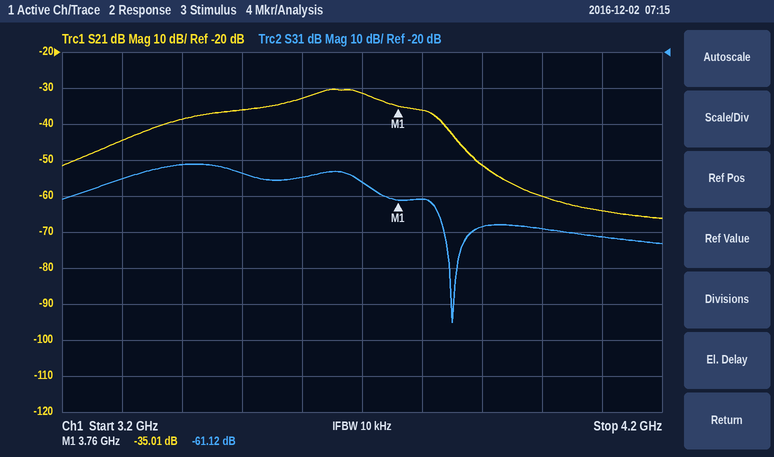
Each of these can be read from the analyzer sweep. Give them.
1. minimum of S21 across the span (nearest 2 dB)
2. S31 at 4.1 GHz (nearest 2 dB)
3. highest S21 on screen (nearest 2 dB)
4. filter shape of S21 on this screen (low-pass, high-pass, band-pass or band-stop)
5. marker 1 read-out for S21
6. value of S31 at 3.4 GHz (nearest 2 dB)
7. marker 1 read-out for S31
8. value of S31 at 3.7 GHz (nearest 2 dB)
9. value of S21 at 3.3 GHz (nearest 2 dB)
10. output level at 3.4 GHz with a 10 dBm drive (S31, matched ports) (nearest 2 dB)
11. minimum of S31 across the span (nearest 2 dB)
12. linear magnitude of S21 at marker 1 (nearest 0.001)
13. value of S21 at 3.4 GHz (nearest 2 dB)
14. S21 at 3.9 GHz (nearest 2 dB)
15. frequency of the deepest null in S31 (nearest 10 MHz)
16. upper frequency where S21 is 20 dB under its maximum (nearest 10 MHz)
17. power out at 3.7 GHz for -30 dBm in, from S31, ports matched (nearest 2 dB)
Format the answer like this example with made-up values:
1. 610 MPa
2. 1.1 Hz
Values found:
1. -66 dB
2. -72 dB
3. -30 dB
4. band-pass
5. -35.01 dB
6. -52 dB
7. -61.12 dB
8. -56 dB
9. -44 dB
10. -42 dBm
11. -96 dB
12. 0.018
13. -38 dB
14. -52 dB
15. 3.85 GHz
16. 3.89 GHz
17. -86 dBm
